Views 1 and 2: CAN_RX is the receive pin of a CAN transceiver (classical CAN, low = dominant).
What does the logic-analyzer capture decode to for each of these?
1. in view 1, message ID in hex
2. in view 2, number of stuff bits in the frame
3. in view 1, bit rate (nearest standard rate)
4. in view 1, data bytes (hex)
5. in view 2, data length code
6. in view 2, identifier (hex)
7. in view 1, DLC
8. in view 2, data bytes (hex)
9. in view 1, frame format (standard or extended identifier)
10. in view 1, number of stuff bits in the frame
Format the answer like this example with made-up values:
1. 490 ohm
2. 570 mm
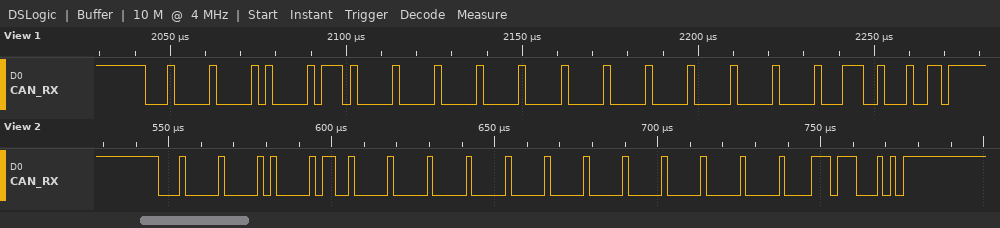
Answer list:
1. 0x100
2. 14
3. 500 kbit/s
4. 1D 00 00 00 00 00 00 00
5. 8
6. 0x100
7. 8
8. 19 00 00 00 00 00 00 00
9. standard
10. 14
